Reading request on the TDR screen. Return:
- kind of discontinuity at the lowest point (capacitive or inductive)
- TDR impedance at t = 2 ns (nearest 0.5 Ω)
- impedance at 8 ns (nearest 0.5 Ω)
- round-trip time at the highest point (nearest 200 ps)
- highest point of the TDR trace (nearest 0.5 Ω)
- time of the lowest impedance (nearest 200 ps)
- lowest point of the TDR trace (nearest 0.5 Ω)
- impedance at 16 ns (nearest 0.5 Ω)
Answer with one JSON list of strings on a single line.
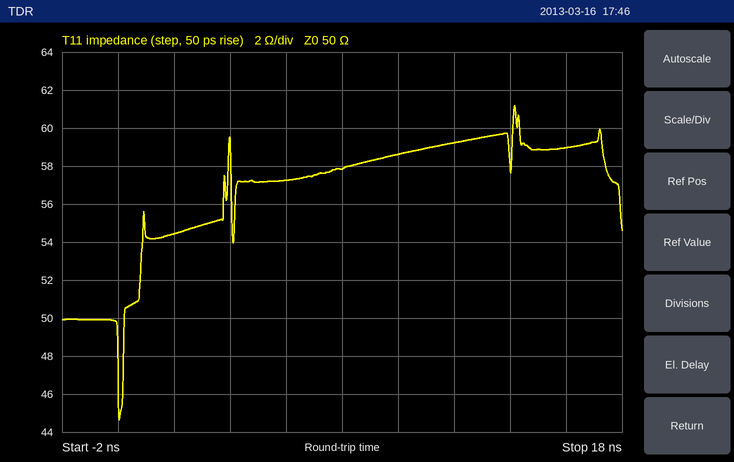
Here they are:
["capacitive", "54.5 Ω", "58.0 Ω", "14.2 ns", "61.0 Ω", "0.0 ns", "44.5 Ω", "59.0 Ω"]
